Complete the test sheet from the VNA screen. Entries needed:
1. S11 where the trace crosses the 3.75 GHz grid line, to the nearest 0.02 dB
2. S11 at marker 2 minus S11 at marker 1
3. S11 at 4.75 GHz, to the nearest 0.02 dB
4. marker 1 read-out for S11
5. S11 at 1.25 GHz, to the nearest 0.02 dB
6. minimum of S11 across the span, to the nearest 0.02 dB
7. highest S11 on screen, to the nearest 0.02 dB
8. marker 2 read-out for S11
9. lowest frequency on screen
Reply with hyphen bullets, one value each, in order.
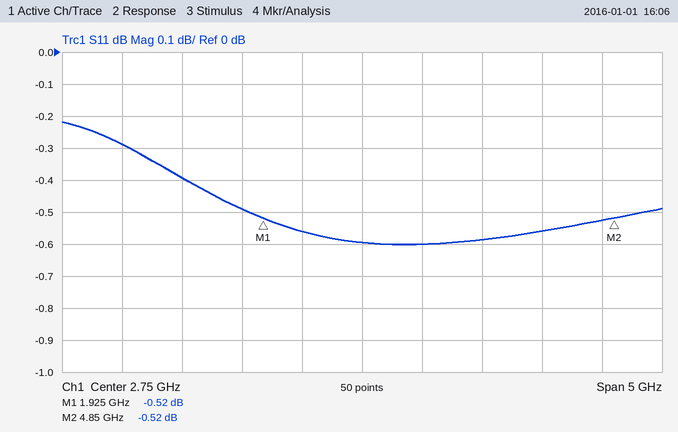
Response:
- -0.58 dB
- 0.00 dB
- -0.52 dB
- -0.52 dB
- -0.40 dB
- -0.60 dB
- -0.22 dB
- -0.52 dB
- 250 MHz
